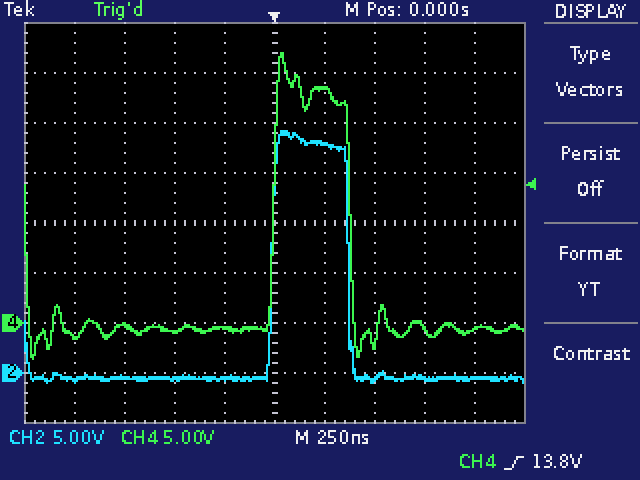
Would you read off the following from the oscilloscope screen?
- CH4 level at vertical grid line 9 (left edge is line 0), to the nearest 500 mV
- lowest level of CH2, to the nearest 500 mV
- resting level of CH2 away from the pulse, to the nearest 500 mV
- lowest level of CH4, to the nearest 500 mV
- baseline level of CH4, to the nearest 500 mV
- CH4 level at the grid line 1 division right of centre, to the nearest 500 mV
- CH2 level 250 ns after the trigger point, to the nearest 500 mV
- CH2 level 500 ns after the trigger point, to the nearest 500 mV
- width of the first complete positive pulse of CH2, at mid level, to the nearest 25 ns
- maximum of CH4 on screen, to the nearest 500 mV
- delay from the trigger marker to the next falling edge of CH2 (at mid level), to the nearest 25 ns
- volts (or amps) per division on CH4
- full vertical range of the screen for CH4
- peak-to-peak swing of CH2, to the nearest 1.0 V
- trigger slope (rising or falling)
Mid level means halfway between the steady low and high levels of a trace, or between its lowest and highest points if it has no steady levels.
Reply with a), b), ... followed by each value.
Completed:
a) -500 mV
b) -1.0 V
c) -500 mV
d) -3.5 V
e) -500 mV
f) 23.5 V
g) 23.0 V
h) -500 mV
i) 375 ns
j) 27.0 V
k) 375 ns
l) 5 V
m) 40 V
n) 25.0 V
o) rising
